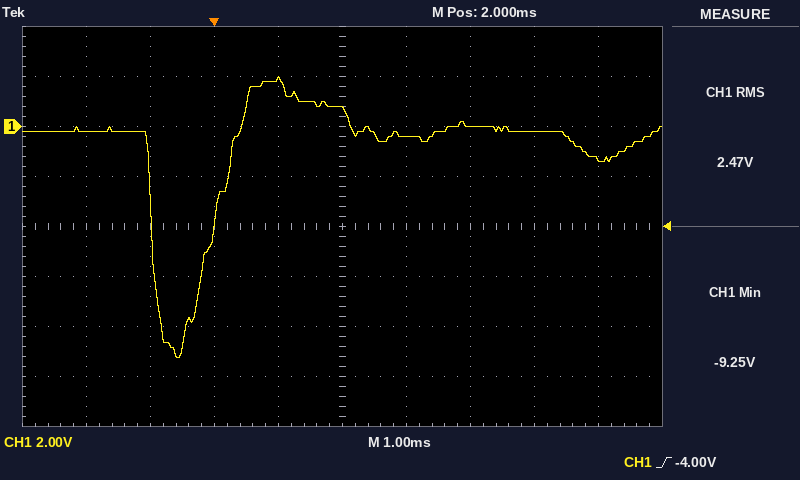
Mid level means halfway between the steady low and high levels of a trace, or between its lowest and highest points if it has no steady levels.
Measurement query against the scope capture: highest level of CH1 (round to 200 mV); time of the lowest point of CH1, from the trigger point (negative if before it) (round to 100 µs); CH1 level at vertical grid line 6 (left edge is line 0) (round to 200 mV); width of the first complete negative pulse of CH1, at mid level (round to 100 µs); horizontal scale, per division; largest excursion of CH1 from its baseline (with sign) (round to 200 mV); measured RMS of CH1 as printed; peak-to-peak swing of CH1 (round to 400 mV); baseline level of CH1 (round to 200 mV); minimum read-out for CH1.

2.0 V
-600 µs
-400 mV
1.0 ms
1 ms
-9.0 V
2.47 V
11.2 V
-200 mV
-9.25 V
